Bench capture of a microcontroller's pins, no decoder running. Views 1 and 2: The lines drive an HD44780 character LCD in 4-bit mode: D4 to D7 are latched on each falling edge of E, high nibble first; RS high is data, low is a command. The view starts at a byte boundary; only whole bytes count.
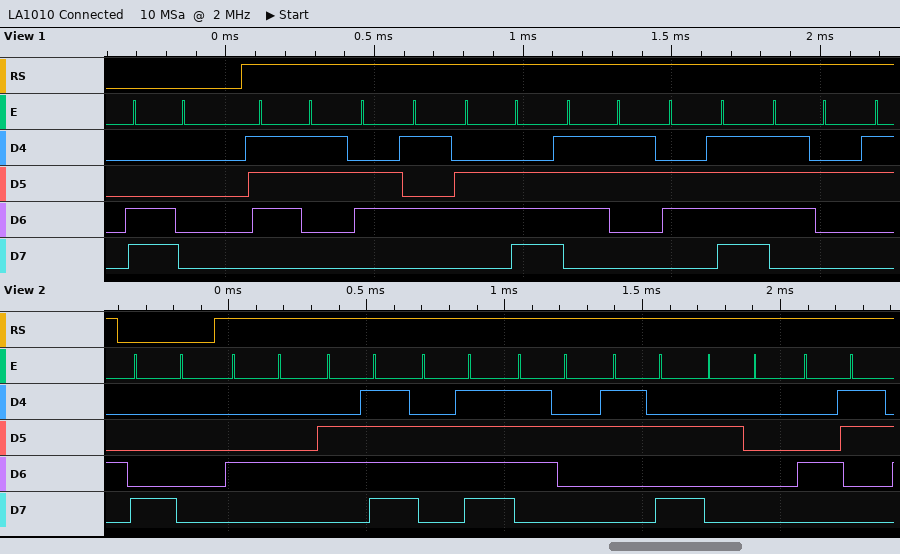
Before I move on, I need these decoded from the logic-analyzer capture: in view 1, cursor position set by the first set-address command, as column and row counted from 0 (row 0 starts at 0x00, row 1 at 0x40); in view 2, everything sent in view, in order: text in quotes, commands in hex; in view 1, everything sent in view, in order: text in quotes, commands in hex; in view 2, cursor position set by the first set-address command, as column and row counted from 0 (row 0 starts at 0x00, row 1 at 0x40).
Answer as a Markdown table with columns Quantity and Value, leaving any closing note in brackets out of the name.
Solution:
| Quantity | Value |
|---|---|
| in view 1, cursor position set by the first set-address command, as column and row counted from 0 | column 0, row 1 |
| in view 2, everything sent in view, in order: text in quotes, commands in hex | 0x80 "Door: C" |
| in view 1, everything sent in view, in order: text in quotes, commands in hex | 0xC0 "sensor" |
| in view 2, cursor position set by the first set-address command, as column and row counted from 0 | column 0, row 0 |
